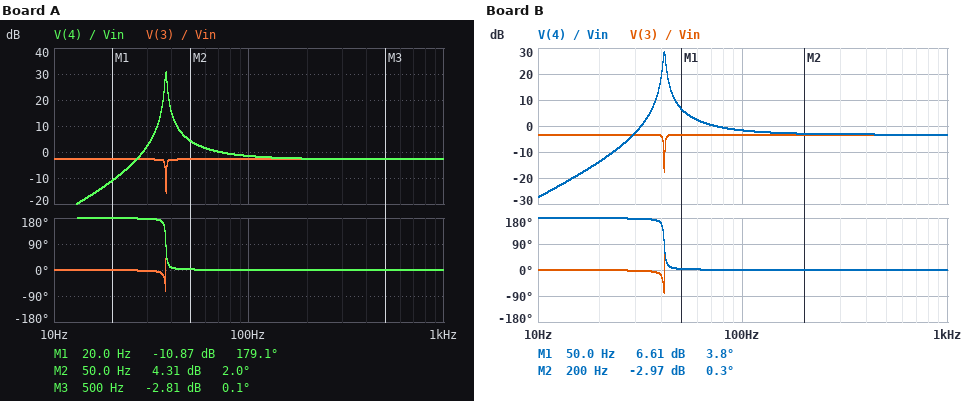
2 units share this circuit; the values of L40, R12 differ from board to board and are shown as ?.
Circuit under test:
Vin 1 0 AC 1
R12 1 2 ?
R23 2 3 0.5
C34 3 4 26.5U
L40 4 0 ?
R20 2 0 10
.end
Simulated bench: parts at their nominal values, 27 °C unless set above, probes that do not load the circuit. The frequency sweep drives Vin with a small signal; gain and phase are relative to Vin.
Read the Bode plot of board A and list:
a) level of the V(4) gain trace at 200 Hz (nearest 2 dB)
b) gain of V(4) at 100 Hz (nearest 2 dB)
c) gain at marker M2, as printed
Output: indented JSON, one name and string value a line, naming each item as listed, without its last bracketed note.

{
  "level of the V(4) gain trace at 200 Hz": "-2 dB",
  "gain of V(4) at 100 Hz": "-2 dB",
  "gain at marker M2, as printed": "4.31 dB"
}
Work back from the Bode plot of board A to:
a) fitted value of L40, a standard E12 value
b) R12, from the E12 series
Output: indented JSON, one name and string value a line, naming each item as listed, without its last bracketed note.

{
  "fitted value of L40, a standard E12 value": "680 mH",
  "R12, from the E12 series": "3.9 Ω"
}
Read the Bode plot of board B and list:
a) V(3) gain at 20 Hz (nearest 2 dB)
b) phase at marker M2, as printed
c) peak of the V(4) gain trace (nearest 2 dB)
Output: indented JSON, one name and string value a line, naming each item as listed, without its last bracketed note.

{
  "V(3) gain at 20 Hz": "-4 dB",
  "phase at marker M2, as printed": "0.3 deg",
  "peak of the V(4) gain trace": "28 dB"
}
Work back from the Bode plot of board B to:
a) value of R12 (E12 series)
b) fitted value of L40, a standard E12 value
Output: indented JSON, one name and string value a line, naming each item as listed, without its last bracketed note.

{
  "value of R12": "4.7 Ω",
  "fitted value of L40, a standard E12 value": "560 mH"
}
